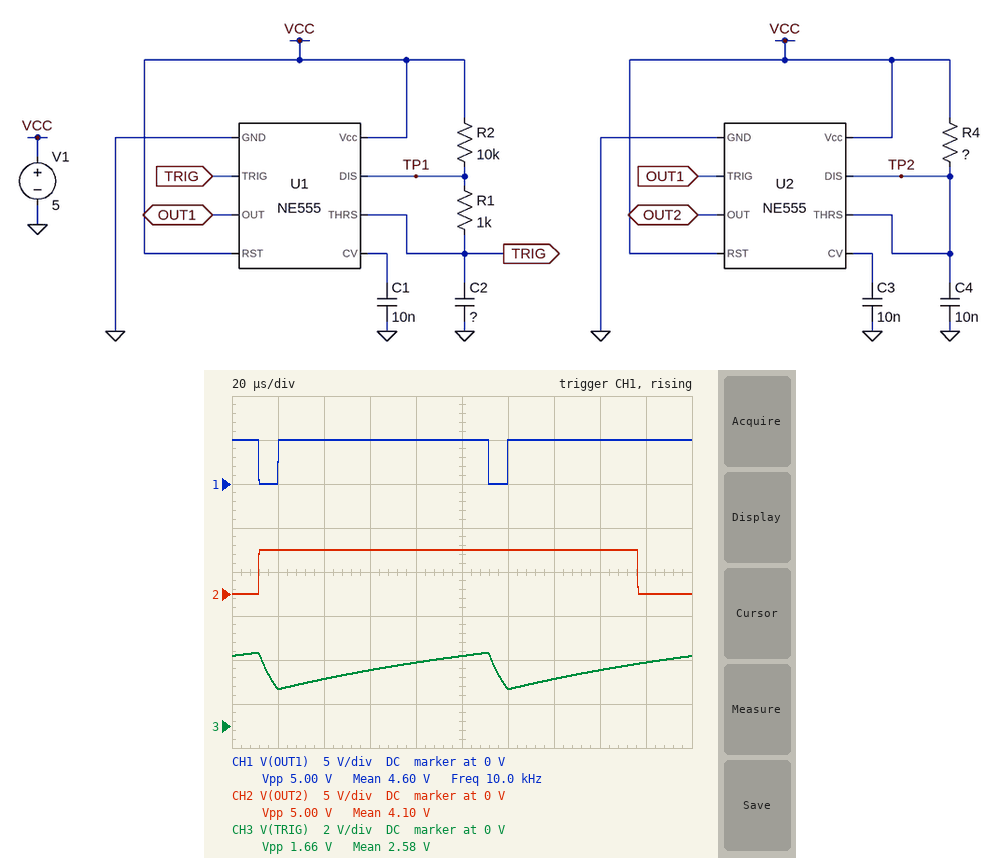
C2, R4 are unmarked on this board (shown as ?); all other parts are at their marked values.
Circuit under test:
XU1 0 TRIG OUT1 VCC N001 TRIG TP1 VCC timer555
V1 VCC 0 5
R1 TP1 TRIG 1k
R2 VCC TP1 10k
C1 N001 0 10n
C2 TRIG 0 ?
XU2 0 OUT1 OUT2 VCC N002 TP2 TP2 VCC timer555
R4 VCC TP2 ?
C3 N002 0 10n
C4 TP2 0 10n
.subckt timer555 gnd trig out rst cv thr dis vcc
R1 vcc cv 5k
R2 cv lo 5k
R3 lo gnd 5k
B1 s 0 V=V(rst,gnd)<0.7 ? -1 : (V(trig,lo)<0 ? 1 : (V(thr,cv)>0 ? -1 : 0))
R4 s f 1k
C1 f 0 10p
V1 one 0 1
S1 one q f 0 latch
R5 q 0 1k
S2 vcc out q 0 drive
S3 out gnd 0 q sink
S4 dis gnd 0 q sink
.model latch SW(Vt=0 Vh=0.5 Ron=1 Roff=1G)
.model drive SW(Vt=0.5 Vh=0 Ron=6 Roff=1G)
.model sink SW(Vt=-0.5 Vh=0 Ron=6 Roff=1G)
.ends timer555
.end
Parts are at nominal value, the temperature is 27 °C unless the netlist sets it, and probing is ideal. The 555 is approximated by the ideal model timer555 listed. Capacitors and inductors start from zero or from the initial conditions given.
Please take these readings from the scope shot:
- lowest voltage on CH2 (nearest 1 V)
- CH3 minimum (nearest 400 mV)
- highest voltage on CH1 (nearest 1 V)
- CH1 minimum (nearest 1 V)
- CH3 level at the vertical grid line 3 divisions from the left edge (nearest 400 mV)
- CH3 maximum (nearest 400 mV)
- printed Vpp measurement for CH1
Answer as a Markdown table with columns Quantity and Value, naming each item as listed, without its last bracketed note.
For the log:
| Quantity | Value |
|---|---|
| lowest voltage on CH2 | 0 V |
| CH3 minimum | 1.6 V |
| highest voltage on CH1 | 5 V |
| CH1 minimum | 0 V |
| CH3 level at the vertical grid line 3 divisions from the left edge | 2.4 V |
| CH3 maximum | 3.2 V |
| printed Vpp measurement for CH1 | 5.00 V |
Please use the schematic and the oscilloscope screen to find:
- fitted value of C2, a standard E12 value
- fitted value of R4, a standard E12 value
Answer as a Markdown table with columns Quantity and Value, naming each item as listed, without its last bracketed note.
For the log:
| Quantity | Value |
|---|---|
| fitted value of C2, a standard E12 value | 12 nF |
| fitted value of R4, a standard E12 value | 15 kΩ |
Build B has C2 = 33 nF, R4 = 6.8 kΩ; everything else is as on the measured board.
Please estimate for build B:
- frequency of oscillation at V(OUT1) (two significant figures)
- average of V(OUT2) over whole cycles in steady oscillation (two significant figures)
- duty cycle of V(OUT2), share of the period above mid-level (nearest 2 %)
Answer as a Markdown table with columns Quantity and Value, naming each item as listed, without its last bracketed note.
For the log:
| Quantity | Value |
|---|---|
| frequency of oscillation at V(OUT1) | 3.6 kHz |
| average of V(OUT2) over whole cycles in steady oscillation | 1.4 V |
| duty cycle of V(OUT2), share of the period above mid-level | 28 % |
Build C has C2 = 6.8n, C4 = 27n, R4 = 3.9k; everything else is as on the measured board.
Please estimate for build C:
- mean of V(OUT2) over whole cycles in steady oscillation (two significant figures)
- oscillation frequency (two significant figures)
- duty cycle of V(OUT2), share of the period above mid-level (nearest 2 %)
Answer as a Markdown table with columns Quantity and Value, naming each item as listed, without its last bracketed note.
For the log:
| Quantity | Value |
|---|---|
| mean of V(OUT2) over whole cycles in steady oscillation | 3.5 V |
| oscillation frequency | 18 kHz |
| duty cycle of V(OUT2), share of the period above mid-level | 70 % |
